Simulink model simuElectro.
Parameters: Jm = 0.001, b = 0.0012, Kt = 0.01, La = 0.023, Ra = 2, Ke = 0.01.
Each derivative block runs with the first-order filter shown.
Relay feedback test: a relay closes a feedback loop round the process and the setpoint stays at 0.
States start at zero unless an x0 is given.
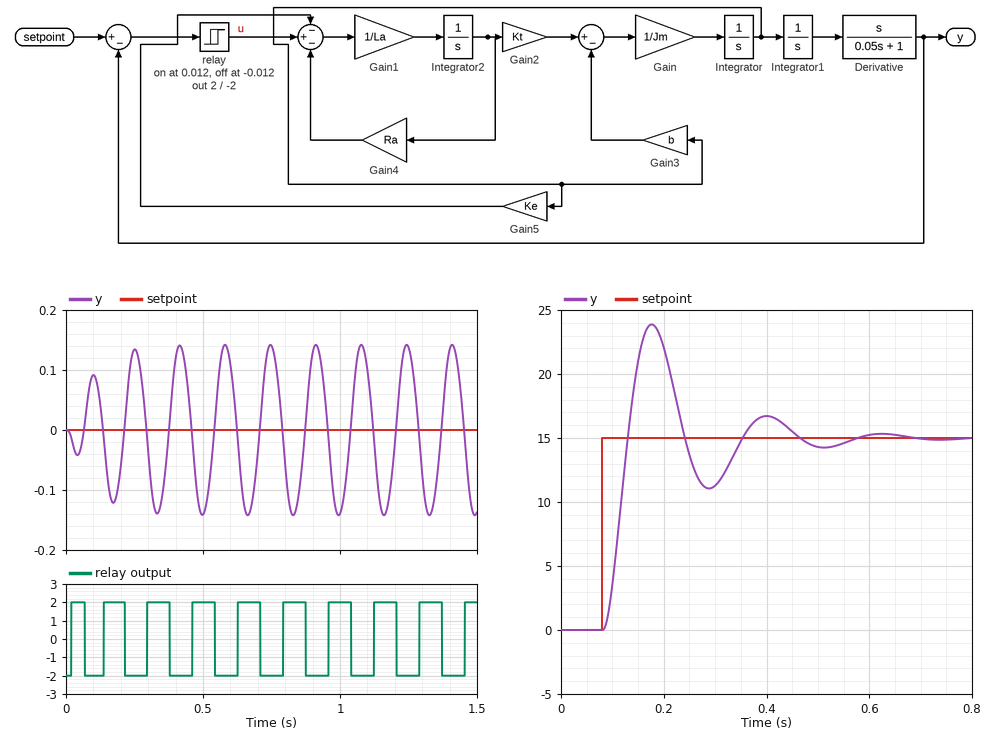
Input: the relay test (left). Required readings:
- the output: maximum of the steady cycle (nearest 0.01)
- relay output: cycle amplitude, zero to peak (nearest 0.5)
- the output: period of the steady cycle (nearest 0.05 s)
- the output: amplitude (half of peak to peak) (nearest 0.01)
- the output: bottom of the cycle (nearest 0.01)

0.14
2.0
0.15 s
0.14
-0.14
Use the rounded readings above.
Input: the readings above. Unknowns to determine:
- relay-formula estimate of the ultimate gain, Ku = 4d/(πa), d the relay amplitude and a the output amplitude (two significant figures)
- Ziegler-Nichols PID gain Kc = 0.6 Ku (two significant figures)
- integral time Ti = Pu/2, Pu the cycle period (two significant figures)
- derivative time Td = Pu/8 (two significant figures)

18
11
0.075 s
0.019 s
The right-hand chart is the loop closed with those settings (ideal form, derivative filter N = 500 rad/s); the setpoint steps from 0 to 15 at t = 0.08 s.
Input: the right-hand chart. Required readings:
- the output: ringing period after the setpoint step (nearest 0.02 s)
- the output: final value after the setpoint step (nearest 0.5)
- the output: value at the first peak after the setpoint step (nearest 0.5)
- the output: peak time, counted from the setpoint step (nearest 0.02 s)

0.22 s
15.0
24.0
0.10 s
